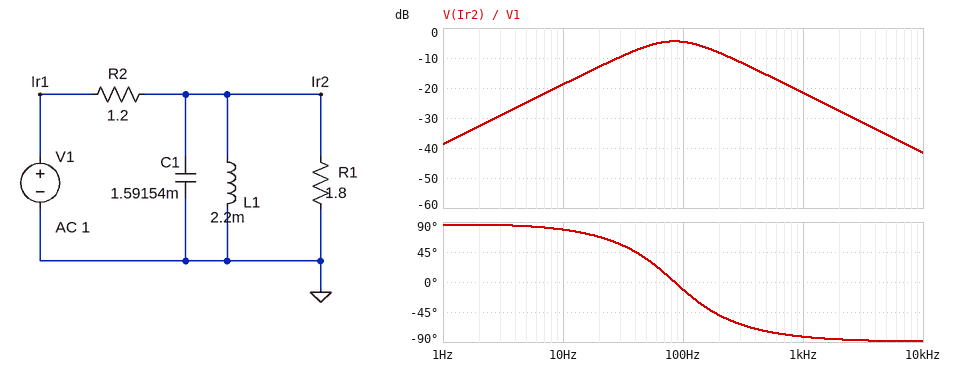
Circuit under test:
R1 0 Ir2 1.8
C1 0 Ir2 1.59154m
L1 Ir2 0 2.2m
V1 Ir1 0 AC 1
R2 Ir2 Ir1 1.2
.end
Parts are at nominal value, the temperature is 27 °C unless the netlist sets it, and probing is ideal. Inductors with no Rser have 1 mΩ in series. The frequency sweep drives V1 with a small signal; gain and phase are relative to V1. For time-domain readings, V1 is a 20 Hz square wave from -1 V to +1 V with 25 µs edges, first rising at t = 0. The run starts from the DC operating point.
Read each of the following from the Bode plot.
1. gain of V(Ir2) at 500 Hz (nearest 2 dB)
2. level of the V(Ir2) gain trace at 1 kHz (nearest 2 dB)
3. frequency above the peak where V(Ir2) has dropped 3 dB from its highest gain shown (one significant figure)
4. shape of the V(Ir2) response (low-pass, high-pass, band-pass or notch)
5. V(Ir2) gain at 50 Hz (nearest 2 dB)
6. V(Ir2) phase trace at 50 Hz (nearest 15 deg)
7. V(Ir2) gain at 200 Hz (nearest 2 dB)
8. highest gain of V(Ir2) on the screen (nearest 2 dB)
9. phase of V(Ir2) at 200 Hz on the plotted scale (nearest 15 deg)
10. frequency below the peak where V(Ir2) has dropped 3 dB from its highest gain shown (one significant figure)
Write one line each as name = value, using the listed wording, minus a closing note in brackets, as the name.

gain of V(Ir2) at 500 Hz = -16 dB
level of the V(Ir2) gain trace at 1 kHz = -22 dB
frequency above the peak where V(Ir2) has dropped 3 dB from its highest gain shown = 200 Hz
shape of the V(Ir2) response = band-pass
V(Ir2) gain at 50 Hz = -6 dB
V(Ir2) phase trace at 50 Hz = 30 deg
V(Ir2) gain at 200 Hz = -8 dB
highest gain of V(Ir2) on the screen = -4 dB
phase of V(Ir2) at 200 Hz on the plotted scale = -45 deg
frequency below the peak where V(Ir2) has dropped 3 dB from its highest gain shown = 40 Hz
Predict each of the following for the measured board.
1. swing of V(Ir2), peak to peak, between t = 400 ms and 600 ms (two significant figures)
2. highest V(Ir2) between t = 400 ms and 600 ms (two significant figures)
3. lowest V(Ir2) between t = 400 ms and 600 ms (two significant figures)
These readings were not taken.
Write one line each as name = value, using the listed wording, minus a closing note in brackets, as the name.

swing of V(Ir2), peak to peak, between t = 400 ms and 600 ms = 1.6 V
highest V(Ir2) between t = 400 ms and 600 ms = 820 mV
lowest V(Ir2) between t = 400 ms and 600 ms = -820 mV
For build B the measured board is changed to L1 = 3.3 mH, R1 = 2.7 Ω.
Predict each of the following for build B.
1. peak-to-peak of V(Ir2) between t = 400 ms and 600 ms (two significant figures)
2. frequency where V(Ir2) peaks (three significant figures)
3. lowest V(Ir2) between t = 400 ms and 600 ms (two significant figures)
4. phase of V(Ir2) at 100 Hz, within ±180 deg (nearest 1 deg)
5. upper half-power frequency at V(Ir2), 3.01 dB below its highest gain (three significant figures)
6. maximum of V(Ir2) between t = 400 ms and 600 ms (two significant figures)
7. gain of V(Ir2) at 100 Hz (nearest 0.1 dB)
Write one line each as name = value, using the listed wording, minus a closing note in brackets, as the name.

peak-to-peak of V(Ir2) between t = 400 ms and 600 ms = 1.9 V
frequency where V(Ir2) peaks = 69.5 Hz
lowest V(Ir2) between t = 400 ms and 600 ms = -970 mV
phase of V(Ir2) at 100 Hz, within ±180 deg = -23 deg
upper half-power frequency at V(Ir2), 3.01 dB below its highest gain = 152 Hz
maximum of V(Ir2) between t = 400 ms and 600 ms = 970 mV
gain of V(Ir2) at 100 Hz = -3.9 dB
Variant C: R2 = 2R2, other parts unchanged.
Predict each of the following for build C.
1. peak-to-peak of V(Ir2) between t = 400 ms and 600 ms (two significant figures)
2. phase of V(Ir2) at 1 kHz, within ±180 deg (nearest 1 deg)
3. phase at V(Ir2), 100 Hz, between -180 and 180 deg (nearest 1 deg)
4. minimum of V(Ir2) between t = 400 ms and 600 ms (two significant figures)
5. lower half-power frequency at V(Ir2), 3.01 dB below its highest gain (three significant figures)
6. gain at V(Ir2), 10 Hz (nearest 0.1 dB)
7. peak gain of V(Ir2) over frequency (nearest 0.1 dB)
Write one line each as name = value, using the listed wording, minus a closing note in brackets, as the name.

peak-to-peak of V(Ir2) between t = 400 ms and 600 ms = 1.1 V
phase of V(Ir2) at 1 kHz, within ±180 deg = -84 deg
phase at V(Ir2), 100 Hz, between -180 and 180 deg = -15 deg
minimum of V(Ir2) between t = 400 ms and 600 ms = -540 mV
lower half-power frequency at V(Ir2), 3.01 dB below its highest gain = 48.4 Hz
gain at V(Ir2), 10 Hz = -24.0 dB
peak gain of V(Ir2) over frequency = -6.9 dB
